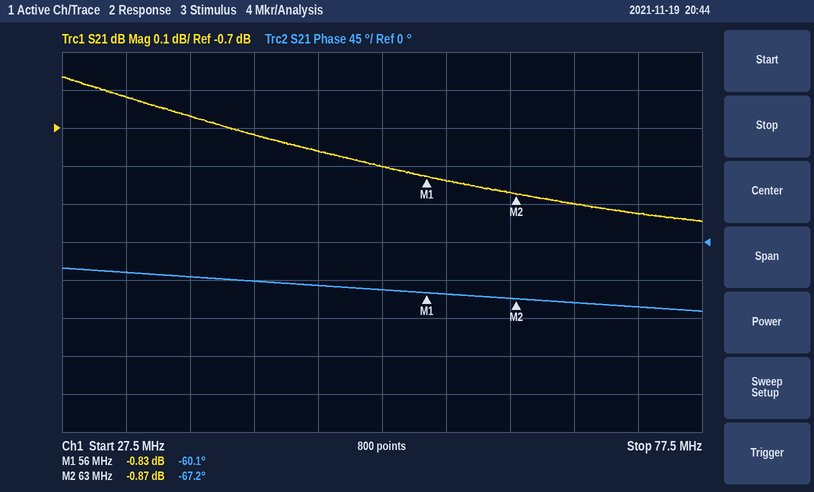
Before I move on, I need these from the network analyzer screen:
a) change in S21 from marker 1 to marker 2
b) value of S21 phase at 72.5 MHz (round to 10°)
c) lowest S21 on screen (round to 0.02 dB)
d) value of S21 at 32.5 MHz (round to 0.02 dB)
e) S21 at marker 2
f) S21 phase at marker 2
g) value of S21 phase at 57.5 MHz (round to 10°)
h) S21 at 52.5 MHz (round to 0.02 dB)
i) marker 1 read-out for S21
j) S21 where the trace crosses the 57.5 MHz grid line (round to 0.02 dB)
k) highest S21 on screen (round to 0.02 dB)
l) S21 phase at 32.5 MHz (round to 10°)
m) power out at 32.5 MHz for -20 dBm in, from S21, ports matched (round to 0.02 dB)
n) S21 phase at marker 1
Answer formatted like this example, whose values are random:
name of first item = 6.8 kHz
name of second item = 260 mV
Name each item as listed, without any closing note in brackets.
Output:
change in S21 from marker 1 to marker 2 = -0.04 dB
value of S21 phase at 72.5 MHz = -80°
lowest S21 on screen = -0.94 dB
value of S21 at 32.5 MHz = -0.62 dB
S21 at marker 2 = -0.87 dB
S21 phase at marker 2 = -67.2°
value of S21 phase at 57.5 MHz = -60°
S21 at 52.5 MHz = -0.80 dB
marker 1 read-out for S21 = -0.83 dB
S21 where the trace crosses the 57.5 MHz grid line = -0.84 dB
highest S21 on screen = -0.56 dB
S21 phase at 32.5 MHz = -40°
power out at 32.5 MHz for -20 dBm in, from S21, ports matched = -20.62 dBm
S21 phase at marker 1 = -60.1°
